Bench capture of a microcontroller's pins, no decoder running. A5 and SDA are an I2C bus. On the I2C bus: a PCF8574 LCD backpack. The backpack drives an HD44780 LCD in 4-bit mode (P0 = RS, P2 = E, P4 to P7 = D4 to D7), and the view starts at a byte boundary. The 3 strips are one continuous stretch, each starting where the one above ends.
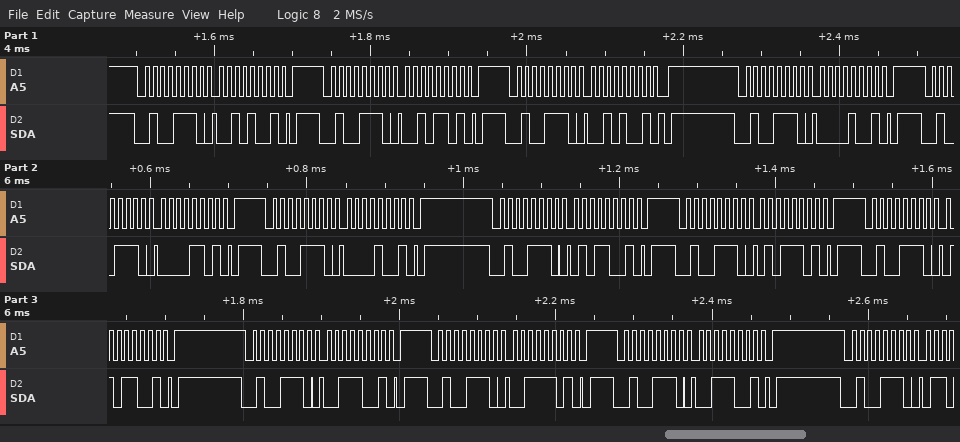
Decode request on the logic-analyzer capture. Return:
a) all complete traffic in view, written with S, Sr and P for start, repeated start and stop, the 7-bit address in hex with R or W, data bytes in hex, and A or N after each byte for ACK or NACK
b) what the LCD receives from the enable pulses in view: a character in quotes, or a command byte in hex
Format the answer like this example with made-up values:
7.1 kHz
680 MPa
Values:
S 27W A 29 A P S 27W A 2D A P S 27W A 29 A P S 27W A 09 A P S 27W A 0D A P S 27W A 09 A P S 27W A 59 A P S 27W A 5D A P S 27W A 59 A P S 27W A 39 A P S 27W A 3D A P S 27W A 39 A P S 27W A
' ' 'S'
